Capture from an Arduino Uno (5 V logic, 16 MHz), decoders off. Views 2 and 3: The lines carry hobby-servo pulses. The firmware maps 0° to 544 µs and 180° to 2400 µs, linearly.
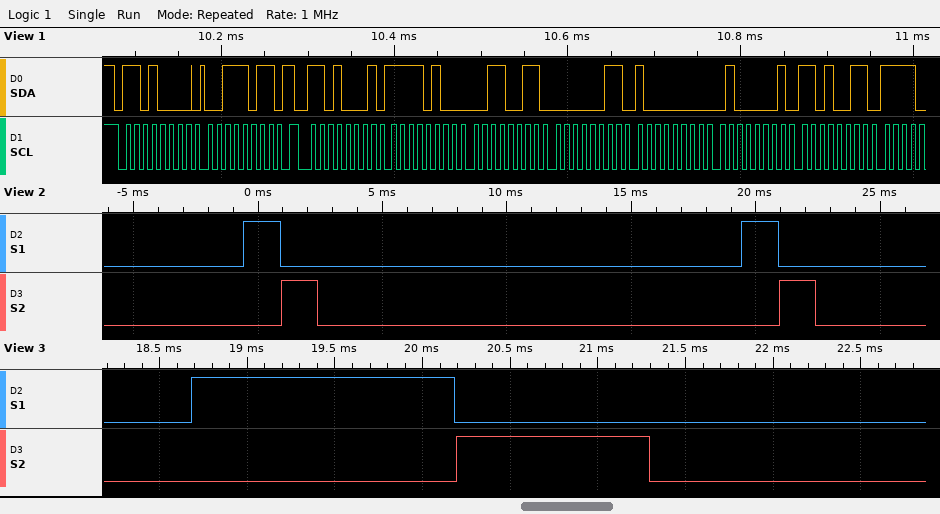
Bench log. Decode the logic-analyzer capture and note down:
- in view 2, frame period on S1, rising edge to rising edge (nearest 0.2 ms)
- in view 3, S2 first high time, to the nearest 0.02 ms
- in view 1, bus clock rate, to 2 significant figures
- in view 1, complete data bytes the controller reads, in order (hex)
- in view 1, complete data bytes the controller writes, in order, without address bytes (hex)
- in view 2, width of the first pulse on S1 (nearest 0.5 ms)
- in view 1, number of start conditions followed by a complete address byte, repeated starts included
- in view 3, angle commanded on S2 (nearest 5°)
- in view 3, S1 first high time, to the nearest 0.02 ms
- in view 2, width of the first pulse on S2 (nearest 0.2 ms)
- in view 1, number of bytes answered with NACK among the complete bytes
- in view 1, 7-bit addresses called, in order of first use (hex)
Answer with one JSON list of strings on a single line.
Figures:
["20.0 ms", "1.10 ms", "100 kHz", "F4 33 03 80 41 D3", "3B", "1.5 ms", "2", "55°", "1.50 ms", "1.4 ms", "0", "0x68"]
